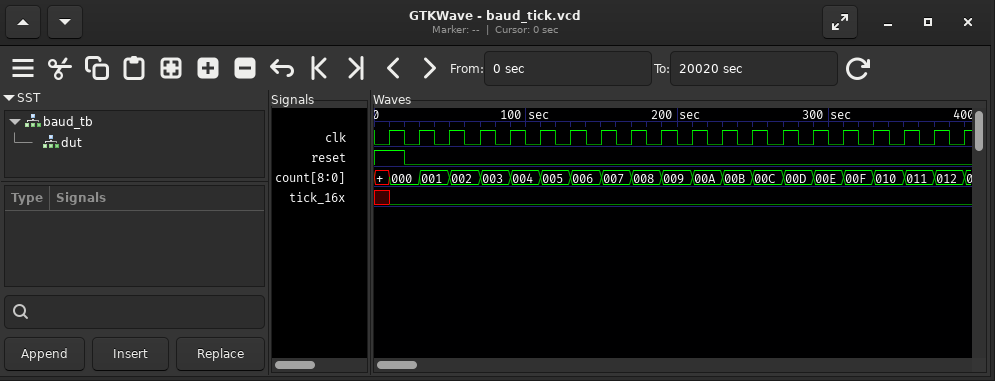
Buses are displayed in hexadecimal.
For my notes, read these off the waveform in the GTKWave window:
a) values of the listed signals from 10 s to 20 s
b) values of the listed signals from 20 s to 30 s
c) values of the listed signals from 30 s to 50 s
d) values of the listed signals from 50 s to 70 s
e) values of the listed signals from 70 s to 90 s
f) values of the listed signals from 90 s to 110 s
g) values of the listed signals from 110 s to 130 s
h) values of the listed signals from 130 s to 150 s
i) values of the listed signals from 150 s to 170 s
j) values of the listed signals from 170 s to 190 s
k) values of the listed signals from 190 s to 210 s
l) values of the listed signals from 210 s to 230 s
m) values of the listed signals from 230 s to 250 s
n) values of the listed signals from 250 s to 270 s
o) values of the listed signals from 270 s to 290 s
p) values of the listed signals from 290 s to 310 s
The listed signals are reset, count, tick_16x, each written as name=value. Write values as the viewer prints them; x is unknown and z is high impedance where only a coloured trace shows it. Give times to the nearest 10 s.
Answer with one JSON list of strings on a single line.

["reset=1, count=000, tick_16x=0", "reset=0, count=000, tick_16x=0", "reset=0, count=001, tick_16x=0", "reset=0, count=002, tick_16x=0", "reset=0, count=003, tick_16x=0", "reset=0, count=004, tick_16x=0", "reset=0, count=005, tick_16x=0", "reset=0, count=006, tick_16x=0", "reset=0, count=007, tick_16x=0", "reset=0, count=008, tick_16x=0", "reset=0, count=009, tick_16x=0", "reset=0, count=00A, tick_16x=0", "reset=0, count=00B, tick_16x=0", "reset=0, count=00C, tick_16x=0", "reset=0, count=00D, tick_16x=0", "reset=0, count=00E, tick_16x=0"]
